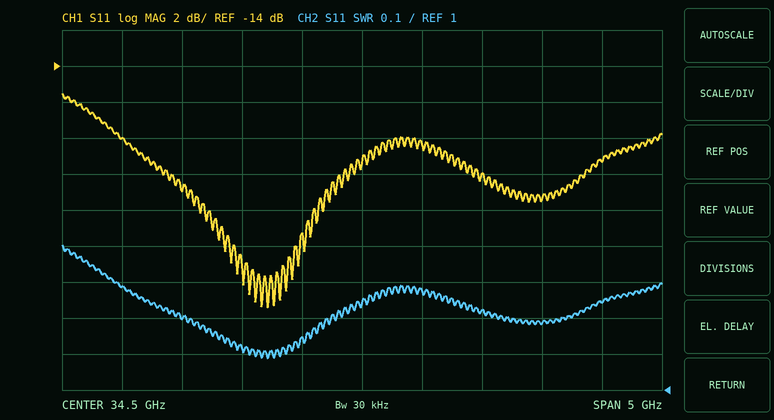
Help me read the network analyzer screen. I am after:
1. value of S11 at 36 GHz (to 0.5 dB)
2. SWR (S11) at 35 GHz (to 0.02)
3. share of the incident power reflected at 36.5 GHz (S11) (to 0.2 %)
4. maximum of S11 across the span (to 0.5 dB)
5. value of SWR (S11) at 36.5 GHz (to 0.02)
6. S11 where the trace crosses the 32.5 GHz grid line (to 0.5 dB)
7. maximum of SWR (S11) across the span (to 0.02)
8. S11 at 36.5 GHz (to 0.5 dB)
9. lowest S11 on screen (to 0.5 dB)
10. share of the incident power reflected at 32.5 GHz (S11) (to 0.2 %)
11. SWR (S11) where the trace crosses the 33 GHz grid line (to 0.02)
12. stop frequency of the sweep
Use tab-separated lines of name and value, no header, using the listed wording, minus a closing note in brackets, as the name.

value of S11 at 36 GHz	-21.5 dB
SWR (S11) at 35 GHz	1.28
share of the incident power reflected at 36.5 GHz (S11)	1.2 %
maximum of S11 across the span	-15.5 dB
value of SWR (S11) at 36.5 GHz	1.24
S11 where the trace crosses the 32.5 GHz grid line	-18.0 dB
maximum of SWR (S11) across the span	1.40
S11 at 36.5 GHz	-19.5 dB
lowest S11 on screen	-27.5 dB
share of the incident power reflected at 32.5 GHz (S11)	1.6 %
SWR (S11) where the trace crosses the 33 GHz grid line	1.20
stop frequency of the sweep	37 GHz
